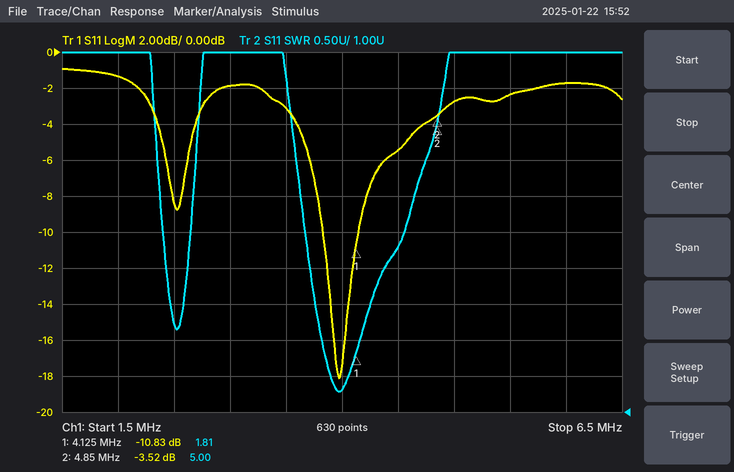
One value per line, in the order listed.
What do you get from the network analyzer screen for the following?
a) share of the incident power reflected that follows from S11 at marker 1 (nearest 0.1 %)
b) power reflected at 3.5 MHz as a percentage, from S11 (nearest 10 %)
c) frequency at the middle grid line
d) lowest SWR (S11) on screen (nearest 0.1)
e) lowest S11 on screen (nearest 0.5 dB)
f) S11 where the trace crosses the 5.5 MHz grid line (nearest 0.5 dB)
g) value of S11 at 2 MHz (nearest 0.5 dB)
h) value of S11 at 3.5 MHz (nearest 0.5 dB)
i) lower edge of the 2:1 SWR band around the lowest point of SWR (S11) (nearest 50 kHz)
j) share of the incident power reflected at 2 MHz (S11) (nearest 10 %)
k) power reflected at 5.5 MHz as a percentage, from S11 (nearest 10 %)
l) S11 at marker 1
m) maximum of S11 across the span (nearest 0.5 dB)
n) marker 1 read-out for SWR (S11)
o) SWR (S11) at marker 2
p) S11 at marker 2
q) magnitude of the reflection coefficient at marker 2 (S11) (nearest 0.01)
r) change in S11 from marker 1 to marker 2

8.3 %
50 %
4 MHz
1.3
-18.0 dB
-2.5 dB
-1.5 dB
-3.0 dB
3.80 MHz
70 %
60 %
-10.83 dB
-1.0 dB
1.81
5.00
-3.52 dB
0.67
7.31 dB
